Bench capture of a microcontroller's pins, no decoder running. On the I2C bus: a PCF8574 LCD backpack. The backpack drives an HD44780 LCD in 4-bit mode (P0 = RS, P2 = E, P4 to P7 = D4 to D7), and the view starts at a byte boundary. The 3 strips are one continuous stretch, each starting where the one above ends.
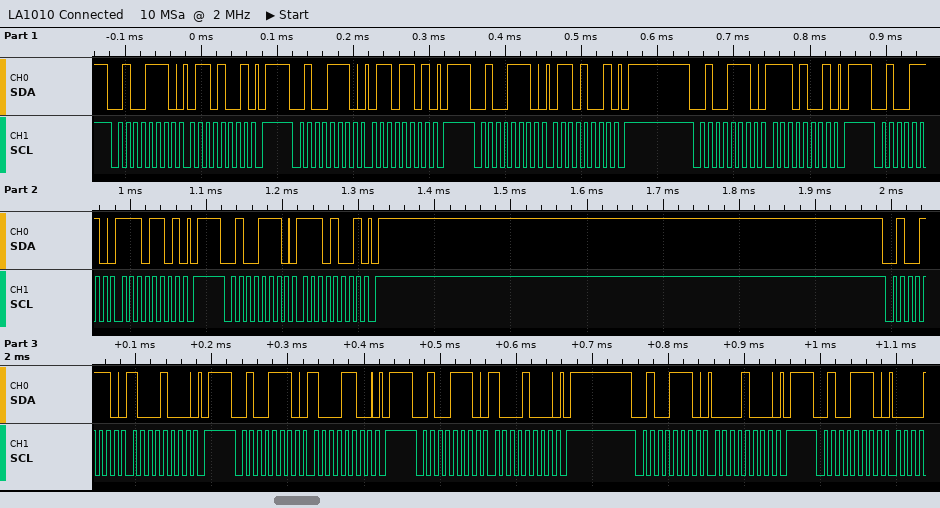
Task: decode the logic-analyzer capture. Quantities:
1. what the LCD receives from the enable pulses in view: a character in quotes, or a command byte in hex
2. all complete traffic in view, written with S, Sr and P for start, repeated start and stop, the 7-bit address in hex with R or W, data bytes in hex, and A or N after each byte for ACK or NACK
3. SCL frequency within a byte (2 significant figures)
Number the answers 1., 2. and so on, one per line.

1. 'n'
2. S 27W A 69 A P S 27W A 6D A P S 27W A 69 A P S 27W A E9 A P S 27W A ED A P S 27W A E9 A P S 27W A 88 A P S 27W A 8C A P S 27W A 88 A P S 27W A 08 A P S 27W A
3. 100 kHz
